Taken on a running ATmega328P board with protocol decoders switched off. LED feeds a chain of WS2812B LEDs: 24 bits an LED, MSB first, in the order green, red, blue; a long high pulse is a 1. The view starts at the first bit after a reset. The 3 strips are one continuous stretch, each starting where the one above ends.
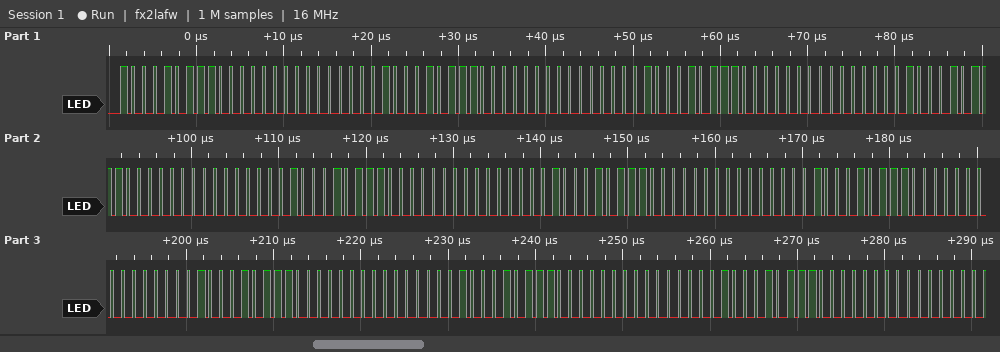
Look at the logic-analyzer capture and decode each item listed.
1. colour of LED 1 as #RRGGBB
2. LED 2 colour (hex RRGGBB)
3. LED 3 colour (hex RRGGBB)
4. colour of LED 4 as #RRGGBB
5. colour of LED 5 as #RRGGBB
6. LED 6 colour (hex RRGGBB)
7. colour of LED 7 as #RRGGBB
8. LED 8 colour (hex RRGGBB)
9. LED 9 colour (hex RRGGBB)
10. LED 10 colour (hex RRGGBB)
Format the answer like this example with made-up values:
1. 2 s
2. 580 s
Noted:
1. #808B00
2. #808B00
3. #808B00
4. #808B00
5. #808B00
6. #808B00
7. #808B00
8. #808B00
9. #808B00
10. #808B00
